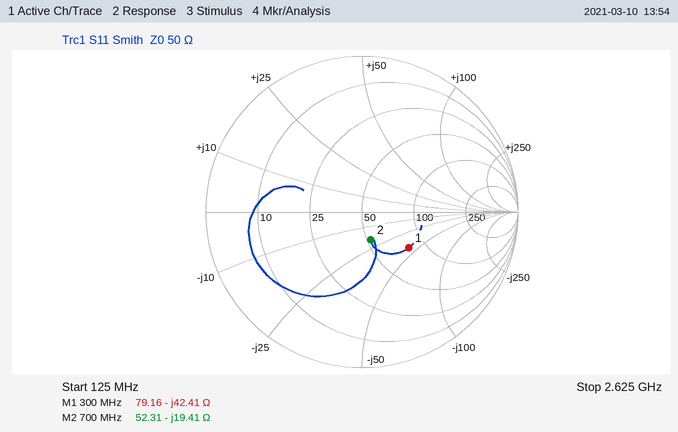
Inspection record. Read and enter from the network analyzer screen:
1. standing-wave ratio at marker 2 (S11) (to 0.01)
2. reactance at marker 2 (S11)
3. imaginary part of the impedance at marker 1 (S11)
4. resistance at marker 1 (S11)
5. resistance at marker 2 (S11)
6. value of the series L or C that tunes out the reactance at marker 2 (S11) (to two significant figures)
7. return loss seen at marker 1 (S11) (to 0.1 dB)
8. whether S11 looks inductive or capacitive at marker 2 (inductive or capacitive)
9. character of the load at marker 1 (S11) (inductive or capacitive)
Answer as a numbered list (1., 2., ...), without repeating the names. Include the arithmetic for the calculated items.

1. 1.46
2. -19.41 Ω
3. -42.41 Ω
4. 79.16 Ω
5. 52.31 Ω
6. L = 19.41 Ω/(2π × 700 MHz) ≈ 4.4 nH
7. 8.4 dB
8. capacitive
9. capacitive
